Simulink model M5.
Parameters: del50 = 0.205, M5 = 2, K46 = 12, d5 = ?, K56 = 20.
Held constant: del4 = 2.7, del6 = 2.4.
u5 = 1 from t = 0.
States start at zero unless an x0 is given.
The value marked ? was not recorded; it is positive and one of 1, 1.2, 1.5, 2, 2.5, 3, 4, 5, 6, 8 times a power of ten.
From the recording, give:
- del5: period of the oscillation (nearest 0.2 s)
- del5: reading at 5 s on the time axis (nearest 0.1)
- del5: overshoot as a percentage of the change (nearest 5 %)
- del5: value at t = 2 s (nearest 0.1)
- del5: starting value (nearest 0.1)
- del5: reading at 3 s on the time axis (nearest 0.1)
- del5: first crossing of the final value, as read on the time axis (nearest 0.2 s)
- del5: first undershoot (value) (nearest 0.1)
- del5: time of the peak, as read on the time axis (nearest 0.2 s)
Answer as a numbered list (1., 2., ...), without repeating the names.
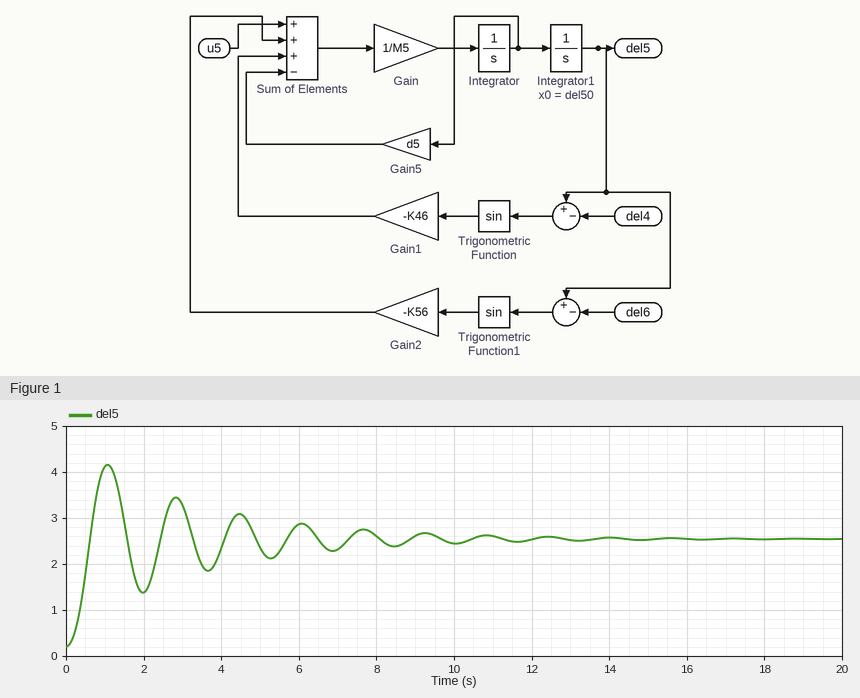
1. 1.8 s
2. 2.4
3. 70 %
4. 1.4
5. 0.2
6. 3.3
7. 0.6 s
8. 1.4
9. 1.0 s
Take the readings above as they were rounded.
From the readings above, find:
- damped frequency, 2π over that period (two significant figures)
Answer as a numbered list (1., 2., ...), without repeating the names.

1. 3.5 rad/s
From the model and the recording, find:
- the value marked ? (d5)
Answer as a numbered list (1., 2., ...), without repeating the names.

1. 1.2
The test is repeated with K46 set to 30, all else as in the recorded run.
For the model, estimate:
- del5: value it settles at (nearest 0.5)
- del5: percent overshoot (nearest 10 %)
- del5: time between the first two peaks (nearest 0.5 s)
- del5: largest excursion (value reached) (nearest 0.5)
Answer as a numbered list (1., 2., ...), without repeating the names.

1. 2.5
2. 70 %
3. 1.5 s
4. 4.5
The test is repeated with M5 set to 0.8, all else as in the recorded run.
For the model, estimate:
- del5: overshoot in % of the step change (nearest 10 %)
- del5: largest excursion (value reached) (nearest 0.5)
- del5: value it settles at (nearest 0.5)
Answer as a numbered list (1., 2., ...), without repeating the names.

1. 60 %
2. 4.0
3. 2.5
